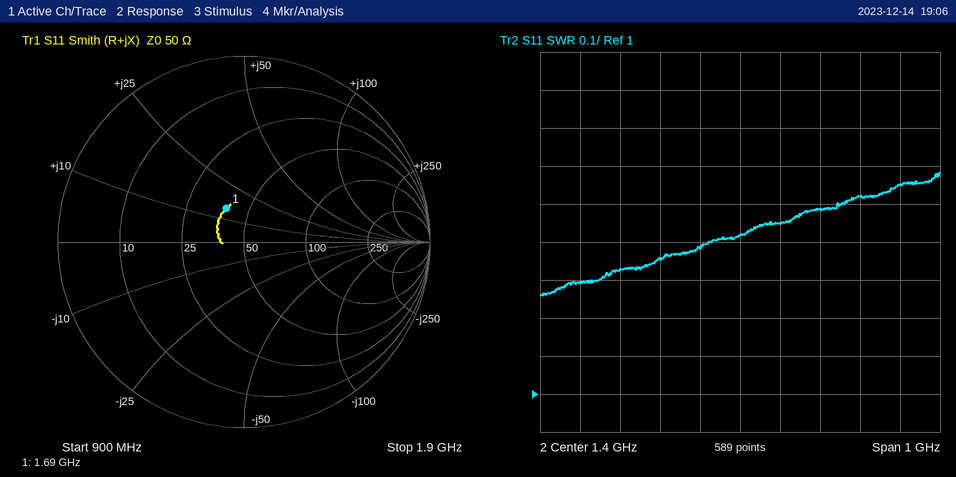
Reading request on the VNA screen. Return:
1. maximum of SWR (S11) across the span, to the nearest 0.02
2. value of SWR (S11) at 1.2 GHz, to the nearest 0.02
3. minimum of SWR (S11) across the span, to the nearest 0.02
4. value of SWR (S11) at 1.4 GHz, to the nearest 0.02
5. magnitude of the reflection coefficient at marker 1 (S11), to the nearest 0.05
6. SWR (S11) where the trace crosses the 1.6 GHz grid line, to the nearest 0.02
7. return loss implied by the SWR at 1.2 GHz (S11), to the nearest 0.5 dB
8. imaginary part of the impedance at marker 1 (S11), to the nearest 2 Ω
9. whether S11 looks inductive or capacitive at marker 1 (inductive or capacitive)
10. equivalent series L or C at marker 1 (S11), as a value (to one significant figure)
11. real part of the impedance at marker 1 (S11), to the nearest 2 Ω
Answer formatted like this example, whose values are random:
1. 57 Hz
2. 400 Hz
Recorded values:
1. 1.58
2. 1.36
3. 1.26
4. 1.42
5. 0.20
6. 1.48
7. 16.5 dB
8. +14 Ω
9. inductive
10. 1 nH
11. 38 Ω
